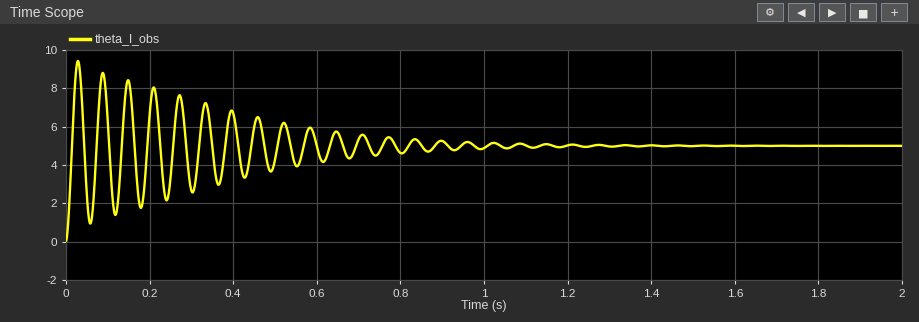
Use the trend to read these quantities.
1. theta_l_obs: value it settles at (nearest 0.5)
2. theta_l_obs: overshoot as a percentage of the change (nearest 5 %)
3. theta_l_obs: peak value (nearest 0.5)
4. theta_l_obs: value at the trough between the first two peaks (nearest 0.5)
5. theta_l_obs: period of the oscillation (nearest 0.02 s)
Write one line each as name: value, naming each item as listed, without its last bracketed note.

theta_l_obs: value it settles at: 5.0
theta_l_obs: overshoot as a percentage of the change: 90 %
theta_l_obs: peak value: 9.5
theta_l_obs: value at the trough between the first two peaks: 1.0
theta_l_obs: period of the oscillation: 0.06 s
